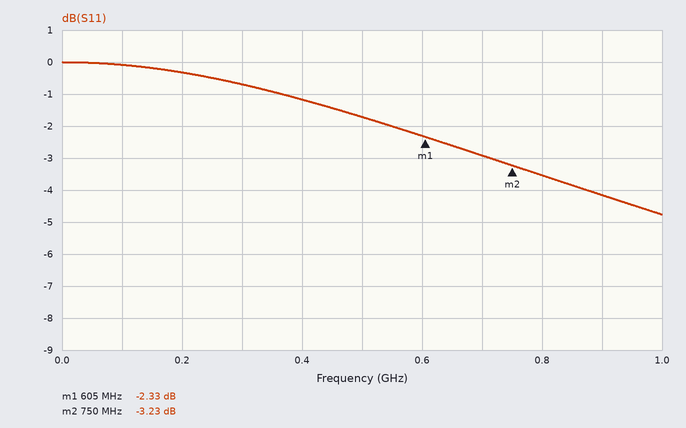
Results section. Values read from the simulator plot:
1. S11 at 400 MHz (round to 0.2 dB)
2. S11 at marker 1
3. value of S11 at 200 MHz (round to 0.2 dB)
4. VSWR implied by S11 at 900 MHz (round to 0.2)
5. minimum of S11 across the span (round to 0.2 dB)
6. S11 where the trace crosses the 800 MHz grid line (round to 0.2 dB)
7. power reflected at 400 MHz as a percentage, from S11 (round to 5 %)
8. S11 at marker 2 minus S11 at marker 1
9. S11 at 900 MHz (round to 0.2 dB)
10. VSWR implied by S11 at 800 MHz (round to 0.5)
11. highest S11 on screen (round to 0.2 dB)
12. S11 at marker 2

-1.2 dB
-2.33 dB
-0.4 dB
4.2
-4.8 dB
-3.6 dB
75 %
-0.90 dB
-4.2 dB
5.0
0.0 dB
-3.23 dB
